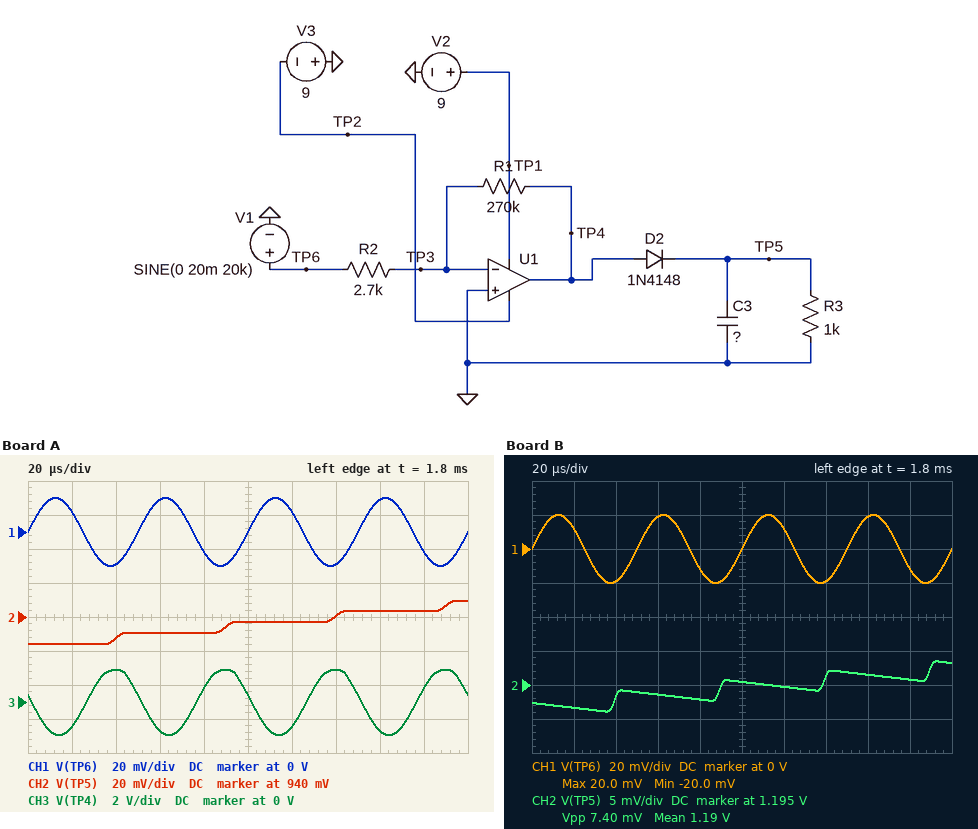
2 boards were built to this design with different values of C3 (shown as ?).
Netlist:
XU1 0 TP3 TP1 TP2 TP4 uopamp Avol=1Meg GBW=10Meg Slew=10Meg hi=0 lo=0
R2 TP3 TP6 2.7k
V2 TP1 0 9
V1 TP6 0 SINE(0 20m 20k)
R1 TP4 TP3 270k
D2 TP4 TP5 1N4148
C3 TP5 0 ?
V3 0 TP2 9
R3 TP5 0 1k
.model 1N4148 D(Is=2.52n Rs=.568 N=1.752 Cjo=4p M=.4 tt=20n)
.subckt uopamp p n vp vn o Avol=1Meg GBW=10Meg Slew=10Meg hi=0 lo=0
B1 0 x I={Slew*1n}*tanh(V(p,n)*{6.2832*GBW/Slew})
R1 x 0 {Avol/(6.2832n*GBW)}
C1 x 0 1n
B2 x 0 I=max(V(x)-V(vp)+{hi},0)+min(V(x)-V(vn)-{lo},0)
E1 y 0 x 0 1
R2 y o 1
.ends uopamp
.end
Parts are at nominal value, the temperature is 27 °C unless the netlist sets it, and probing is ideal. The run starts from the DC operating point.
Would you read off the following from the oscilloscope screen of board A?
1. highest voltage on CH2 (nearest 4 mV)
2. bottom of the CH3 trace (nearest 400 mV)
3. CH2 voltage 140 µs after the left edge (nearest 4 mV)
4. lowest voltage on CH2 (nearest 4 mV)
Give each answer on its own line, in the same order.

948 mV
-2.0 V
940 mV
924 mV
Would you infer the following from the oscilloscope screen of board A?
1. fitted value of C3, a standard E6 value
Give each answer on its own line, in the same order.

220 µF
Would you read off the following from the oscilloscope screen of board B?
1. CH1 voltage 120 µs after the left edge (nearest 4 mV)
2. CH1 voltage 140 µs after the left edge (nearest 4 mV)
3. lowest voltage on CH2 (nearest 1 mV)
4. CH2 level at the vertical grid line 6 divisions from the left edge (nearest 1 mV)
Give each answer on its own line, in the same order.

12 mV
-20 mV
1.191 V
1.195 V
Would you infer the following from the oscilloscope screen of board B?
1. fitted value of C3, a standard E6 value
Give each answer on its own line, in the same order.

33 µF
